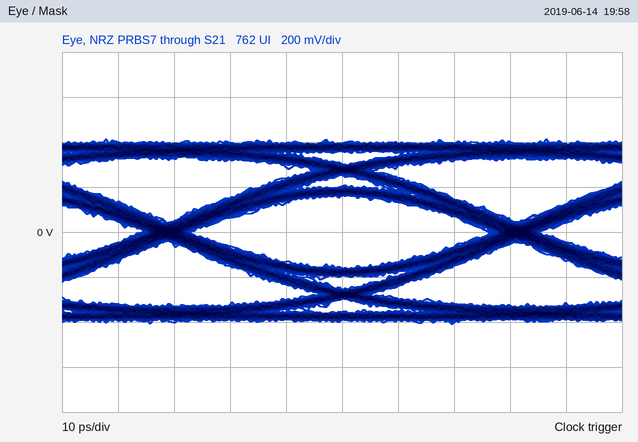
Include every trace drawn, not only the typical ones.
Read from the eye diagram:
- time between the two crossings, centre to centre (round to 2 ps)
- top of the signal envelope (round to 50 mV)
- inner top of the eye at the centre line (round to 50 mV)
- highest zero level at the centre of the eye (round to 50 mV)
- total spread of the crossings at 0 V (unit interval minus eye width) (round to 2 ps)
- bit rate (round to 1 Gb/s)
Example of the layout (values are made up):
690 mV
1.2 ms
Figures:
62 ps
400 mV
150 mV
-150 mV
10 ps
16 Gb/s
